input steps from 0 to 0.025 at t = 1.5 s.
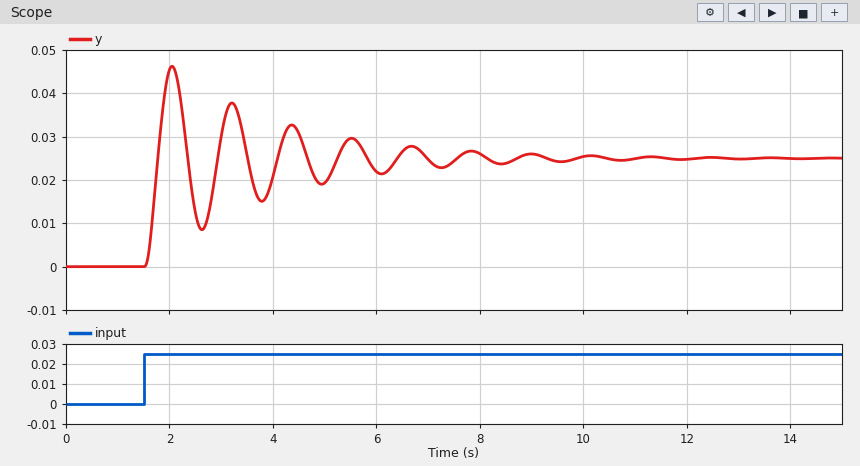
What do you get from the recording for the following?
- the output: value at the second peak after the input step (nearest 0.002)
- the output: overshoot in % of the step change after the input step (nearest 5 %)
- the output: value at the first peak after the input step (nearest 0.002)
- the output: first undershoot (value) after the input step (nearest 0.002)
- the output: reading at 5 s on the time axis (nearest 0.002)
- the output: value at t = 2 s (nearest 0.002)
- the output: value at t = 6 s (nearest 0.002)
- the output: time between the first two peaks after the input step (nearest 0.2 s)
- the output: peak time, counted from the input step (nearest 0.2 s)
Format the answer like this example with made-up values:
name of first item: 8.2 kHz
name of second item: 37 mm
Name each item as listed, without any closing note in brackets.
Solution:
the output: value at the second peak after the input step: 0.038
the output: overshoot in % of the step change after the input step: 85 %
the output: value at the first peak after the input step: 0.046
the output: first undershoot (value) after the input step: 0.008
the output: reading at 5 s on the time axis: 0.020
the output: value at t = 2 s: 0.046
the output: value at t = 6 s: 0.022
the output: time between the first two peaks after the input step: 1.2 s
the output: peak time, counted from the input step: 0.6 s
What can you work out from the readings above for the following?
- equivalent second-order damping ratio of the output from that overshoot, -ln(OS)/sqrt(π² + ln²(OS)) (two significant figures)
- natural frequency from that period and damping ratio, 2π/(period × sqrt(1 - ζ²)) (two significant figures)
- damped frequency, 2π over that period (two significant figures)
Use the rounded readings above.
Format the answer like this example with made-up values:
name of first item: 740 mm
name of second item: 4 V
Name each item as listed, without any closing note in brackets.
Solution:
equivalent second-order damping ratio of the output from that overshoot, -ln(OS)/sqrt(π² + ln²(OS)): 0.052
natural frequency from that period and damping ratio, 2π/(period × sqrt(1 - ζ²)): 5.2 rad/s
damped frequency, 2π over that period: 5.2 rad/s
